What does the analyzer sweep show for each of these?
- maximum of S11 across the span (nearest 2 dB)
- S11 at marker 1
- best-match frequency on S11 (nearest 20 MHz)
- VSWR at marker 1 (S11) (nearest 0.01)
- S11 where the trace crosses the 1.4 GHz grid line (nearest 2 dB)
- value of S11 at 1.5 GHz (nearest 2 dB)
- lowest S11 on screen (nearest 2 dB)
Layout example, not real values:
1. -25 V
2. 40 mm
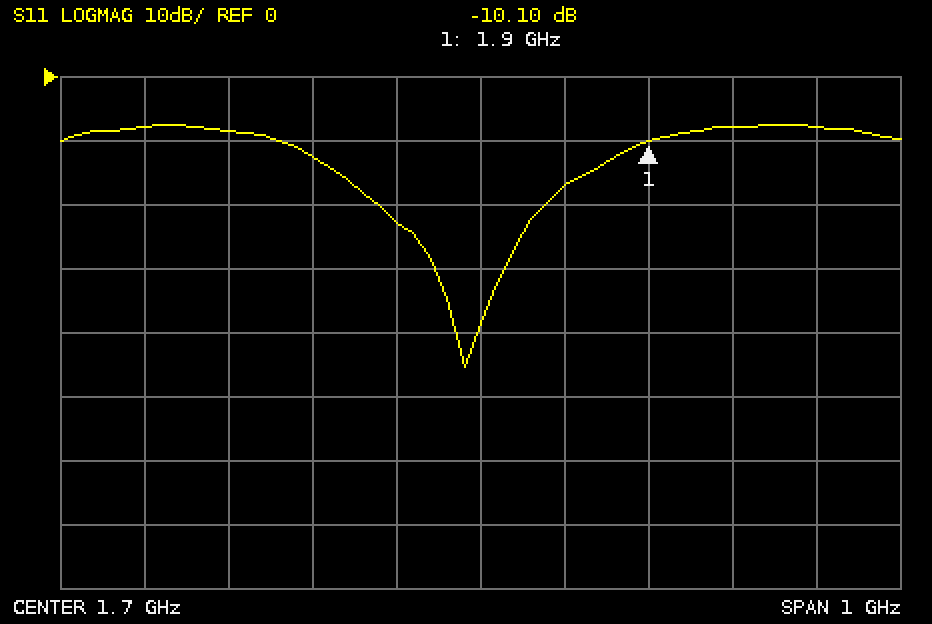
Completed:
1. -8 dB
2. -10.10 dB
3. 1.68 GHz
4. 1.91
5. -8 dB
6. -12 dB
7. -46 dB
